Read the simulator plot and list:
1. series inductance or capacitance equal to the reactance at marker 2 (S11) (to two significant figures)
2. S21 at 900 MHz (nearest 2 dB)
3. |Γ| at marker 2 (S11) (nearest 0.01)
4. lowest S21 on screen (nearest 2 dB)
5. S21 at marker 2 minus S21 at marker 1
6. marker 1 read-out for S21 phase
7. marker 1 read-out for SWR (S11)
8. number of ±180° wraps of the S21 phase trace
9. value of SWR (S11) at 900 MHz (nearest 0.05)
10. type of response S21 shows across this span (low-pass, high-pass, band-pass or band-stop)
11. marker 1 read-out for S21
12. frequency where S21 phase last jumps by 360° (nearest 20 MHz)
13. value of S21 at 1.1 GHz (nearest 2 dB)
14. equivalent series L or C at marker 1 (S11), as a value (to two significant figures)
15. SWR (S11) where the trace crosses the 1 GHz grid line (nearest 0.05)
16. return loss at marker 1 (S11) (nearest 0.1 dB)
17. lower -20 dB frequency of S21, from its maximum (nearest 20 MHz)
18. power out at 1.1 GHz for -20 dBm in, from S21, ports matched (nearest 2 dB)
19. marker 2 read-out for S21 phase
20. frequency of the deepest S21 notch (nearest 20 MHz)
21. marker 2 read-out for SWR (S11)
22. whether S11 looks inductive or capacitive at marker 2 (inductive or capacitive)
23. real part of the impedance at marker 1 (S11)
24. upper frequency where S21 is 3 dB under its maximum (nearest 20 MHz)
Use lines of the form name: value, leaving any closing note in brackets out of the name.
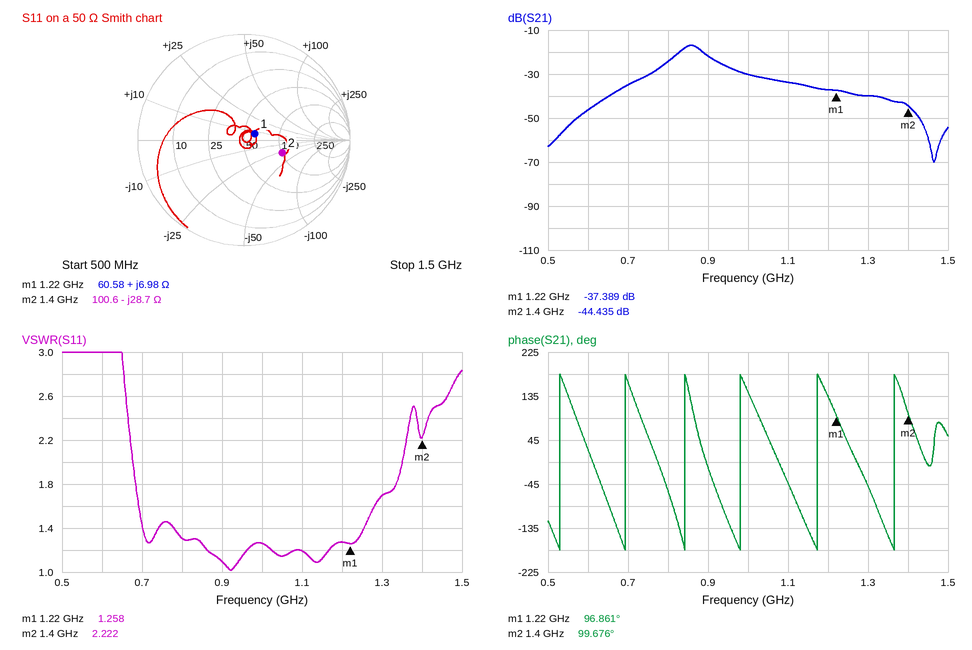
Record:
series inductance or capacitance equal to the reactance at marker 2 (S11): 4.0 pF
S21 at 900 MHz: -22 dB
|Γ| at marker 2 (S11): 0.38
lowest S21 on screen: -70 dB
S21 at marker 2 minus S21 at marker 1: -7.046 dB
marker 1 read-out for S21 phase: 96.861°
marker 1 read-out for SWR: 1.258
number of ±180° wraps of the S21 phase trace: 6
value of SWR (S11) at 900 MHz: 1.10
type of response S21 shows across this span: band-pass
marker 1 read-out for S21: -37.389 dB
frequency where S21 phase last jumps by 360°: 1.36 GHz
value of S21 at 1.1 GHz: -34 dB
equivalent series L or C at marker 1 (S11), as a value: 910 pH
SWR (S11) where the trace crosses the 1 GHz grid line: 1.25
return loss at marker 1 (S11): 18.8 dB
lower -20 dB frequency of S21, from its maximum: 680 MHz
power out at 1.1 GHz for -20 dBm in, from S21, ports matched: -54 dBm
marker 2 read-out for S21 phase: 99.676°
frequency of the deepest S21 notch: 1.46 GHz
marker 2 read-out for SWR: 2.222
whether S11 looks inductive or capacitive at marker 2: capacitive
real part of the impedance at marker 1: 60.58 Ω
upper frequency where S21 is 3 dB under its maximum: 880 MHz
